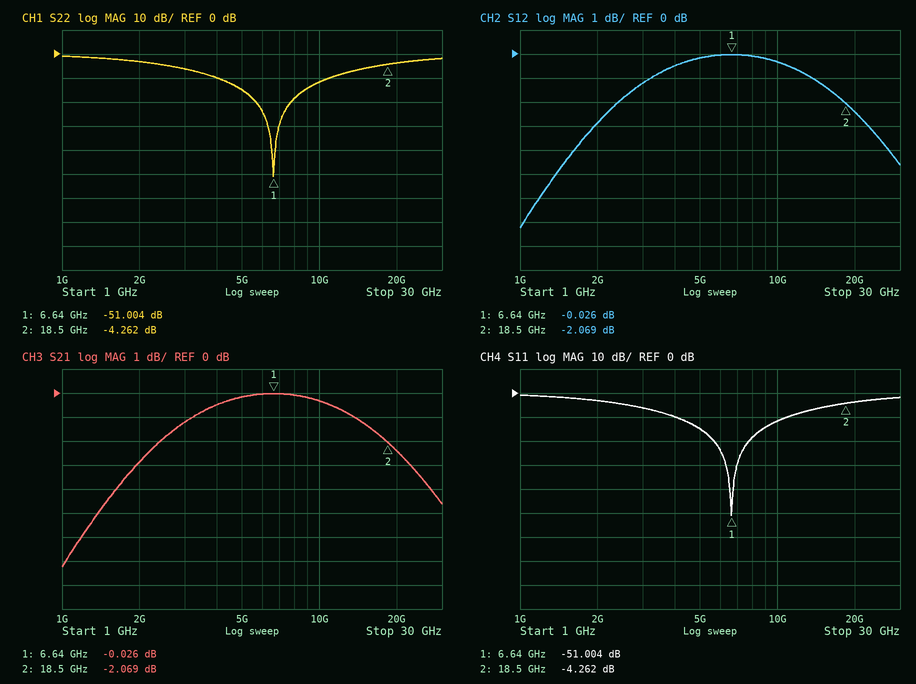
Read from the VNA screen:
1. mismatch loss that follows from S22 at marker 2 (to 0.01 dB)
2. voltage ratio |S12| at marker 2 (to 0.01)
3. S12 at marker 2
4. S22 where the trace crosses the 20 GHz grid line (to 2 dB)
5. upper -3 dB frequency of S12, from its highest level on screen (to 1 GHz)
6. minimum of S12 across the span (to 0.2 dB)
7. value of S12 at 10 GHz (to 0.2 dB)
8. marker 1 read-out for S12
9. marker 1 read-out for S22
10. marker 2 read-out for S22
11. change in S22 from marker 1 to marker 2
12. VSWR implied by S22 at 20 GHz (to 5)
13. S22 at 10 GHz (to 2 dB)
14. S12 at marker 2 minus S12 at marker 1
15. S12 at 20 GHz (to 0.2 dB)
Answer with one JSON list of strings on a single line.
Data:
["2.04 dB", "0.79", "-2.069 dB", "-4 dB", "23 GHz", "-7.2 dB", "-0.4 dB", "-0.026 dB", "-51.004 dB", "-4.262 dB", "46.742 dB", "5", "-12 dB", "-2.043 dB", "-2.4 dB"]
